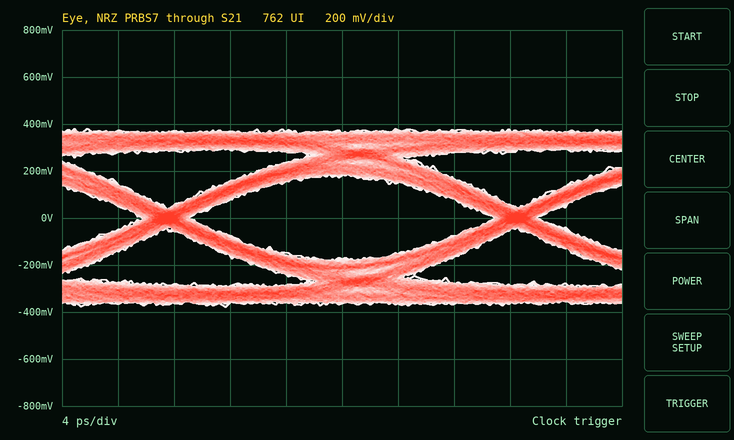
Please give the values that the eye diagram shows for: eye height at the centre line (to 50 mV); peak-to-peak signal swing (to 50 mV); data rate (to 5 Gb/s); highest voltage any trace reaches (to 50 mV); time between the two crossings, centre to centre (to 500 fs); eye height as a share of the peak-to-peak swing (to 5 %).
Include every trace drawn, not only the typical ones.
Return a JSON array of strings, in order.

["350 mV", "750 mV", "40 Gb/s", "400 mV", "25.0 ps", "45 %"]
